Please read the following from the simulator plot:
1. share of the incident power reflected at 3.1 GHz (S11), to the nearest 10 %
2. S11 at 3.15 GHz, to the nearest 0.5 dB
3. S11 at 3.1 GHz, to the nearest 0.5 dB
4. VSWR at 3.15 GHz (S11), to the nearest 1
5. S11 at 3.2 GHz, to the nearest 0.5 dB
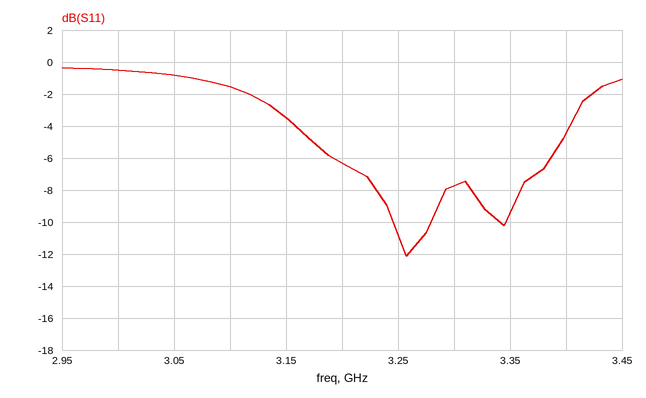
70 %
-3.5 dB
-1.5 dB
5
-6.5 dB
